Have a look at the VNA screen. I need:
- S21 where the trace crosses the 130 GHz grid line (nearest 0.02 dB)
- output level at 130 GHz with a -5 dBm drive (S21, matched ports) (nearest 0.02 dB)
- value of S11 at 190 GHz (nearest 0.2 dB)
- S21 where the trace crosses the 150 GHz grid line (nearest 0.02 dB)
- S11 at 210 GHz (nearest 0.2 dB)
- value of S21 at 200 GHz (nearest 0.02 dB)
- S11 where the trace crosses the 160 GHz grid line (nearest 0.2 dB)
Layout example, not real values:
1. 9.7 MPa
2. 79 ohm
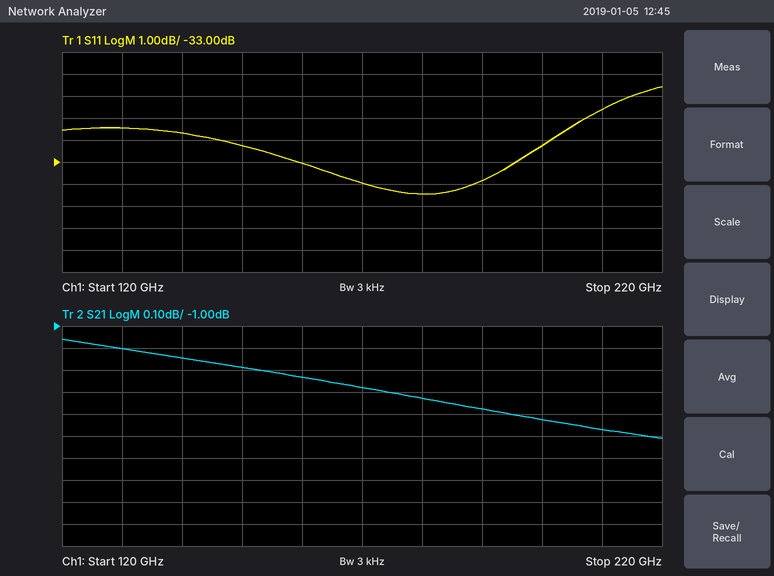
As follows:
1. -1.10 dB
2. -6.10 dBm
3. -33.8 dB
4. -1.18 dB
5. -30.6 dB
6. -1.42 dB
7. -33.0 dB
